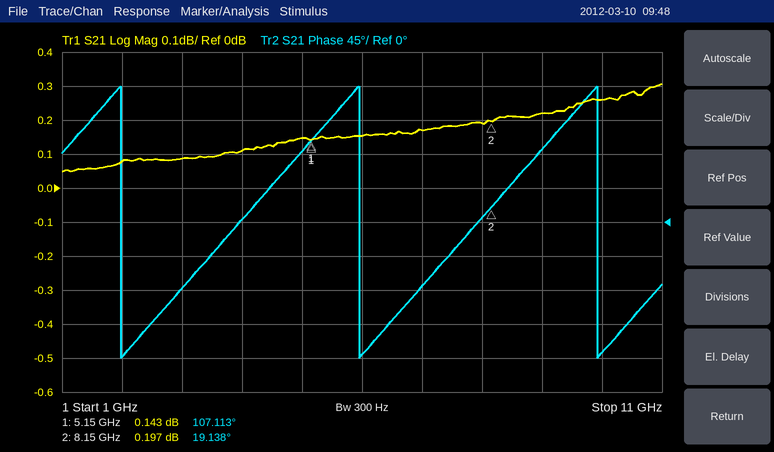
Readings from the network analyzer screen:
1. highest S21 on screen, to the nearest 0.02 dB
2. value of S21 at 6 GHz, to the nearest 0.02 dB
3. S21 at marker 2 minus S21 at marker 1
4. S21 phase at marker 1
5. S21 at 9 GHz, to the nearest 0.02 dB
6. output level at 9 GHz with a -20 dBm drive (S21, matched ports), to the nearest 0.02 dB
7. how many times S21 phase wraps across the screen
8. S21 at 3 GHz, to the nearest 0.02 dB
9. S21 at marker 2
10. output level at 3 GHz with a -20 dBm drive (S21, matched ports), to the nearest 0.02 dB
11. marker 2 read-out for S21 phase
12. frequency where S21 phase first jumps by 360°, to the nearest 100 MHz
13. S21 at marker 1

0.30 dB
0.16 dB
0.054 dB
107.113°
0.22 dB
-19.78 dBm
3
0.08 dB
0.197 dB
-19.92 dBm
19.138°
2.0 GHz
0.143 dB
